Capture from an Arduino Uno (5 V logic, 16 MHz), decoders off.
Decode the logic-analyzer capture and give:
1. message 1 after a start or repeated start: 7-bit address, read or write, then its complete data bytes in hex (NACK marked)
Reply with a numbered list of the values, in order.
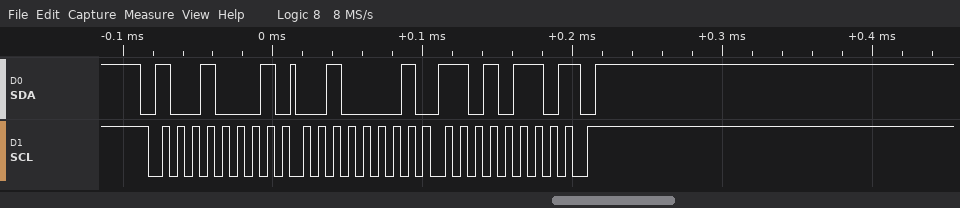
1. 0x48 read: 21 D6 NACK
